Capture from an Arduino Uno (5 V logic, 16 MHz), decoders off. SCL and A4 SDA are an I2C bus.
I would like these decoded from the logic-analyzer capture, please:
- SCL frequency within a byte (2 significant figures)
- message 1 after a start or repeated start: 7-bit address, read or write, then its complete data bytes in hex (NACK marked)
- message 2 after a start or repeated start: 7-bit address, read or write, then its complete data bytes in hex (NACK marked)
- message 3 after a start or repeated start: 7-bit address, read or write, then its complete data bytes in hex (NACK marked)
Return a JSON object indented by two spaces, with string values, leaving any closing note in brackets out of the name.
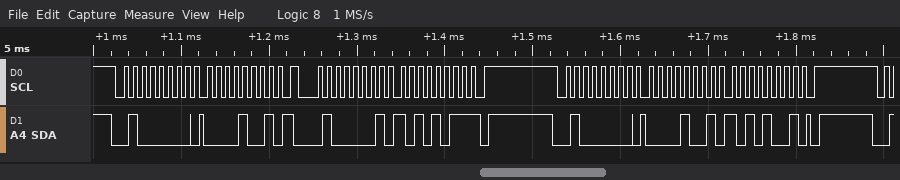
{
  "SCL frequency within a byte": "100 kHz",
  "message 1 after a start or repeated start: 7-bit address, read or write, then its complete data bytes in hex": "0x20 write: 09",
  "message 2 after a start or repeated start: 7-bit address, read or write, then its complete data bytes in hex": "0x20 read: AB NACK",
  "message 3 after a start or repeated start: 7-bit address, read or write, then its complete data bytes in hex": "0x20 write: 09 A9"
}
